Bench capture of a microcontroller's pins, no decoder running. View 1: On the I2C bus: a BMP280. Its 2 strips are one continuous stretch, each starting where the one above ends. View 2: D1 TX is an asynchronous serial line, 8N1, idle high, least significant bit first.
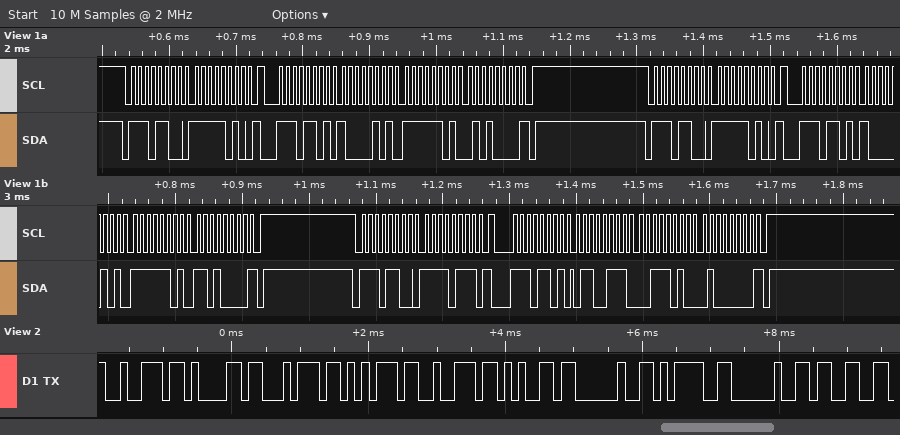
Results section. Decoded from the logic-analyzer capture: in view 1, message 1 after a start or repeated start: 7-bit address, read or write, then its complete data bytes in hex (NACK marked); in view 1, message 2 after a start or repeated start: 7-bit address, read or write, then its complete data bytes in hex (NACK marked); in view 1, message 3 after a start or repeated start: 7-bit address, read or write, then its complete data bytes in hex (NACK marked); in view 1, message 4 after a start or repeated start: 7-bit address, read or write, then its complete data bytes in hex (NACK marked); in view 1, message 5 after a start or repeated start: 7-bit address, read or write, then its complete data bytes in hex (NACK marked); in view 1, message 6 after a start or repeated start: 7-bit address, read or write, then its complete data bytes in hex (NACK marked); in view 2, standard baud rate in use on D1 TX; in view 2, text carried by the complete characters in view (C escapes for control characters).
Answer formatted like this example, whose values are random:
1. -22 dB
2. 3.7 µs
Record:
1. 0x76 write: FA
2. 0x76 read: 85 FD 50 NACK
3. 0x76 write: FA
4. 0x76 read: 85 FD D0 NACK
5. 0x76 write: F7
6. 0x76 read: 67 3A 40 NACK
7. 9600 baud
8. "rature = 3"
